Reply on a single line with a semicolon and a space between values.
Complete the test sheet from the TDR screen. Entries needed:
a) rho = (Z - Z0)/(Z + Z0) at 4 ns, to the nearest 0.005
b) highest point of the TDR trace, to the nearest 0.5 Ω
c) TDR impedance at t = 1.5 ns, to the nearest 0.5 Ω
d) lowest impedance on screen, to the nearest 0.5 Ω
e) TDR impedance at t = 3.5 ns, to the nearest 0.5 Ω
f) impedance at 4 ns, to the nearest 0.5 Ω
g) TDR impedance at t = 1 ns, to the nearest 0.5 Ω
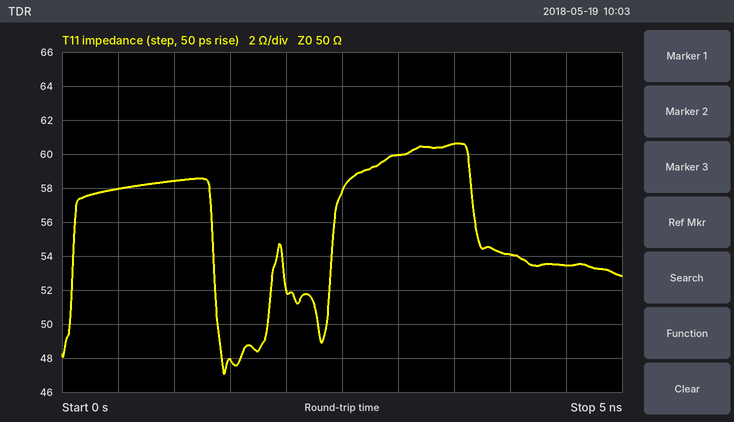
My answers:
+0.040; 60.5 Ω; 48.0 Ω; 47.0 Ω; 60.5 Ω; 54.0 Ω; 58.5 Ω
